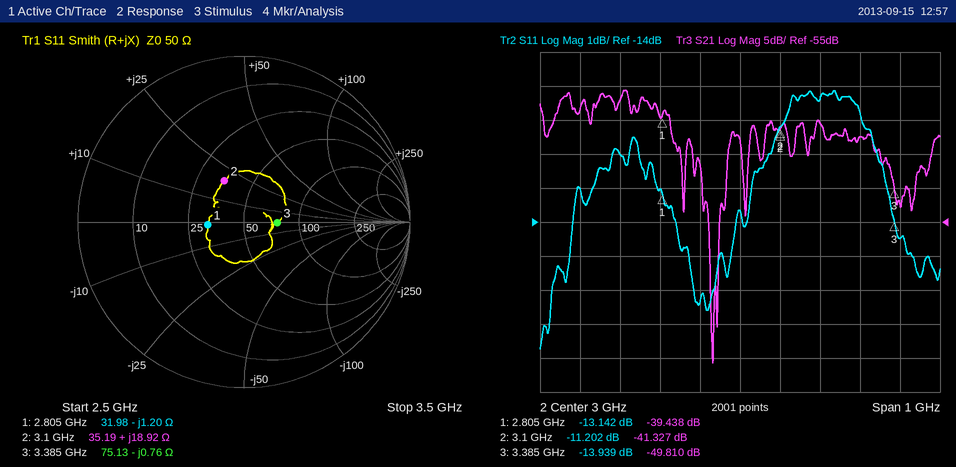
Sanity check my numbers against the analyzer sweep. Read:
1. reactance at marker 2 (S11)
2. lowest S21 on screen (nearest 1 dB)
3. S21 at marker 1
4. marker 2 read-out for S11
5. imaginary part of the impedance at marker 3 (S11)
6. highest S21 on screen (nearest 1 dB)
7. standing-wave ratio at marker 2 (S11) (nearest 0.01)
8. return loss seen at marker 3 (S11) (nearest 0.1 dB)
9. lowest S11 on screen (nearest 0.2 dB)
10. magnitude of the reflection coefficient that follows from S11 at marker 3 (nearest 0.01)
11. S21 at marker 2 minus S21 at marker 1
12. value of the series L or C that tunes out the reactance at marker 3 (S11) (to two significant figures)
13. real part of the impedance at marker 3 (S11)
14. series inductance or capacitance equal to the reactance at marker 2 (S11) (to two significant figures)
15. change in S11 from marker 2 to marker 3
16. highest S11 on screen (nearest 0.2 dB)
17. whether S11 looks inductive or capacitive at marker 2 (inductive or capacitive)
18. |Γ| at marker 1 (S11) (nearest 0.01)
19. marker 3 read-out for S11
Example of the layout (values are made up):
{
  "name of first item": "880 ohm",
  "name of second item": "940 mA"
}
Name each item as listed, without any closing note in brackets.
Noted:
{
  "reactance at marker 2": "+18.92 Ω",
  "lowest S21 on screen": "-76 dB",
  "S21 at marker 1": "-39.438 dB",
  "marker 2 read-out for S11": "-11.202 dB",
  "imaginary part of the impedance at marker 3": "-0.76 Ω",
  "highest S21 on screen": "-36 dB",
  "standing-wave ratio at marker 2 (S11)": "1.76",
  "return loss seen at marker 3 (S11)": "13.9 dB",
  "lowest S11 on screen": "-17.8 dB",
  "magnitude of the reflection coefficient that follows from S11 at marker 3": "0.20",
  "S21 at marker 2 minus S21 at marker 1": "-1.889 dB",
  "value of the series L or C that tunes out the reactance at marker 3 (S11)": "36 pH",
  "real part of the impedance at marker 3": "75.13 Ω",
  "series inductance or capacitance equal to the reactance at marker 2 (S11)": "970 pH",
  "change in S11 from marker 2 to marker 3": "-2.737 dB",
  "highest S11 on screen": "-10.2 dB",
  "whether S11 looks inductive or capacitive at marker 2": "inductive",
  "|Γ| at marker 1 (S11)": "0.22",
  "marker 3 read-out for S11": "-13.939 dB"
}
